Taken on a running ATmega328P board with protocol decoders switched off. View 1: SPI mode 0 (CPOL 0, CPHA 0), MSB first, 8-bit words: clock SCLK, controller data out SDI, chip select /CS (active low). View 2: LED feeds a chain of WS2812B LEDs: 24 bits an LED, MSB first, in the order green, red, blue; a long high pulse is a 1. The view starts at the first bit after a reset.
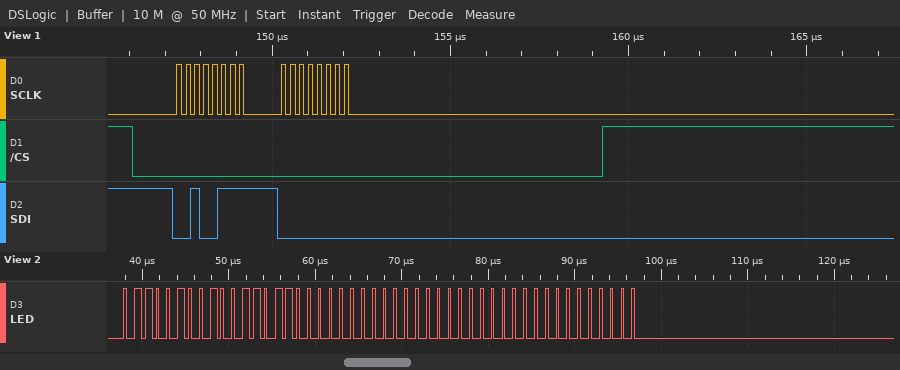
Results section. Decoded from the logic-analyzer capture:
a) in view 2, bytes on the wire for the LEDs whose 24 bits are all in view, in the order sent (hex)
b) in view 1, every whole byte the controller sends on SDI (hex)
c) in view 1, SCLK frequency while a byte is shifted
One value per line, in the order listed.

64 9B 00 00 00 00
27 00
4 MHz
